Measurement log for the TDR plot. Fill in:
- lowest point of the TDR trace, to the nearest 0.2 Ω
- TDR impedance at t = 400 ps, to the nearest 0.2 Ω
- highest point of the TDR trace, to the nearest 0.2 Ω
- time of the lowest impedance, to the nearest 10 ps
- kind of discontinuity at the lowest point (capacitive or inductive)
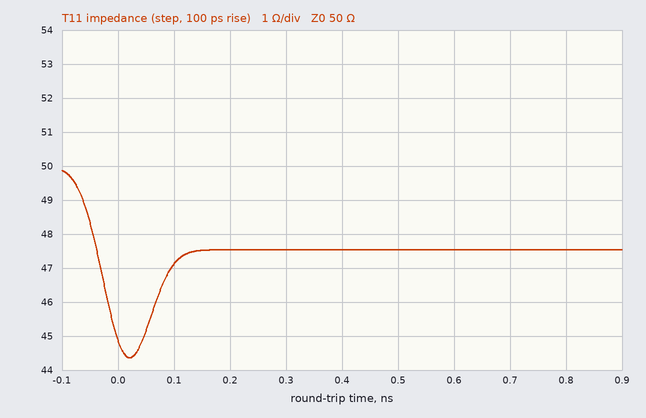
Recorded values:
44.4 Ω
47.6 Ω
49.8 Ω
20 ps
capacitive
